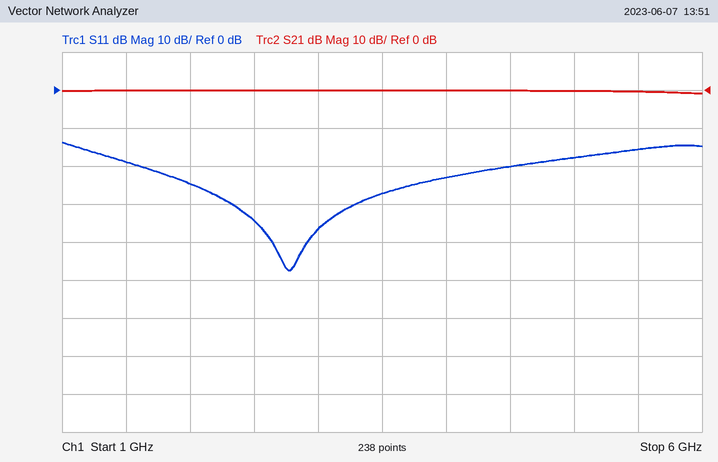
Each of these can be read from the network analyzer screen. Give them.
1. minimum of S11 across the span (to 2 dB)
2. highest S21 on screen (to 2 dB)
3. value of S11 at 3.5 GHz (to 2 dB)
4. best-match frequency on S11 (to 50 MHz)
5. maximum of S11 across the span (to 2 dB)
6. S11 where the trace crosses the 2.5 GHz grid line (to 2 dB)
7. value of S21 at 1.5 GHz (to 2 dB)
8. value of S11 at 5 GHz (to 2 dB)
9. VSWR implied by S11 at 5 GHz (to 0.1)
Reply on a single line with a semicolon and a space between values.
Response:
-48 dB; 0 dB; -28 dB; 2.75 GHz; -14 dB; -34 dB; 0 dB; -18 dB; 1.3
